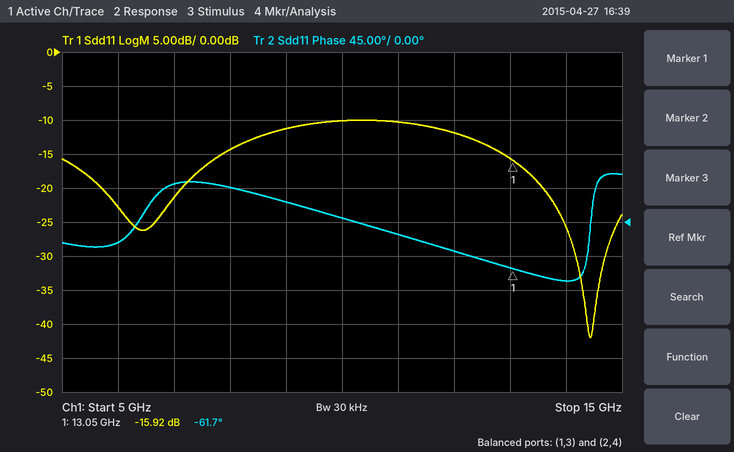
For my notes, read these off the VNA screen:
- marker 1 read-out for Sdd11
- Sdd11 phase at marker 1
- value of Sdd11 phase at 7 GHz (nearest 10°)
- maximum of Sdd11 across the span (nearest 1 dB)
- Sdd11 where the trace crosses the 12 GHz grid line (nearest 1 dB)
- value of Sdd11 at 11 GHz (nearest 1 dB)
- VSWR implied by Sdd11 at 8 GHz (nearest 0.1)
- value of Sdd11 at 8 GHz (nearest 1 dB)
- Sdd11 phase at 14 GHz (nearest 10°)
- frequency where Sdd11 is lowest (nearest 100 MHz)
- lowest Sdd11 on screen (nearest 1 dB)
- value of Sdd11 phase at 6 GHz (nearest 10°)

-15.92 dB
-61.7°
50°
-10 dB
-12 dB
-10 dB
1.5
-14 dB
-80°
14.4 GHz
-42 dB
-30°
